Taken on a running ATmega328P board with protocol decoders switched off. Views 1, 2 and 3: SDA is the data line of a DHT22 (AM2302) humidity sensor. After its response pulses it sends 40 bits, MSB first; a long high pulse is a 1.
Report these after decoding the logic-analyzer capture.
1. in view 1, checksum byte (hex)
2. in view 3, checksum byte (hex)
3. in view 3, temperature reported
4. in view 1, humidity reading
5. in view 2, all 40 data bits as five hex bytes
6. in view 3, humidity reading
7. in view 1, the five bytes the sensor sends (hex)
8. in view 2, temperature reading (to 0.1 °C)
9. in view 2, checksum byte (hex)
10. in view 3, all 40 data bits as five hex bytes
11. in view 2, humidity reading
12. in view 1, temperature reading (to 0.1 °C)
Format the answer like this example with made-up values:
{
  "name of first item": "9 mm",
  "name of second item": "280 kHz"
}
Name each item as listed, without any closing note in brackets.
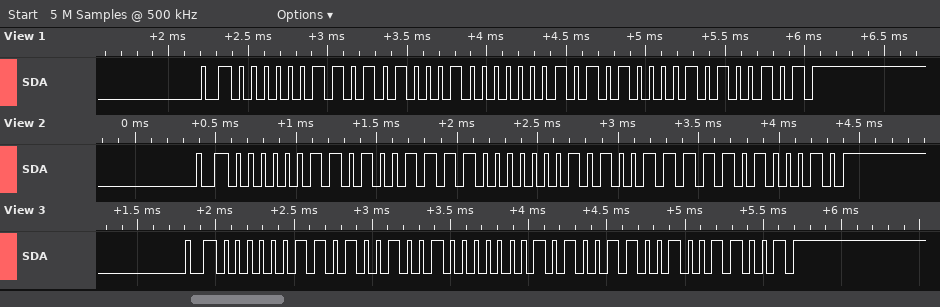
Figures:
{
  "in view 1, checksum byte": "0xA5",
  "in view 3, checksum byte": "0x99",
  "in view 3, temperature reported": "33.2 °C",
  "in view 1, humidity reading": "84.9 %",
  "in view 2, all 40 data bits as five hex bytes": "03 4F 01 4F A2",
  "in view 3, humidity reading": "84.1 %",
  "in view 1, the five bytes the sensor sends": "03 51 01 50 A5",
  "in view 2, temperature reading": "33.5 °C",
  "in view 2, checksum byte": "0xA2",
  "in view 3, all 40 data bits as five hex bytes": "03 49 01 4C 99",
  "in view 2, humidity reading": "84.7 %",
  "in view 1, temperature reading": "33.6 °C"
}
